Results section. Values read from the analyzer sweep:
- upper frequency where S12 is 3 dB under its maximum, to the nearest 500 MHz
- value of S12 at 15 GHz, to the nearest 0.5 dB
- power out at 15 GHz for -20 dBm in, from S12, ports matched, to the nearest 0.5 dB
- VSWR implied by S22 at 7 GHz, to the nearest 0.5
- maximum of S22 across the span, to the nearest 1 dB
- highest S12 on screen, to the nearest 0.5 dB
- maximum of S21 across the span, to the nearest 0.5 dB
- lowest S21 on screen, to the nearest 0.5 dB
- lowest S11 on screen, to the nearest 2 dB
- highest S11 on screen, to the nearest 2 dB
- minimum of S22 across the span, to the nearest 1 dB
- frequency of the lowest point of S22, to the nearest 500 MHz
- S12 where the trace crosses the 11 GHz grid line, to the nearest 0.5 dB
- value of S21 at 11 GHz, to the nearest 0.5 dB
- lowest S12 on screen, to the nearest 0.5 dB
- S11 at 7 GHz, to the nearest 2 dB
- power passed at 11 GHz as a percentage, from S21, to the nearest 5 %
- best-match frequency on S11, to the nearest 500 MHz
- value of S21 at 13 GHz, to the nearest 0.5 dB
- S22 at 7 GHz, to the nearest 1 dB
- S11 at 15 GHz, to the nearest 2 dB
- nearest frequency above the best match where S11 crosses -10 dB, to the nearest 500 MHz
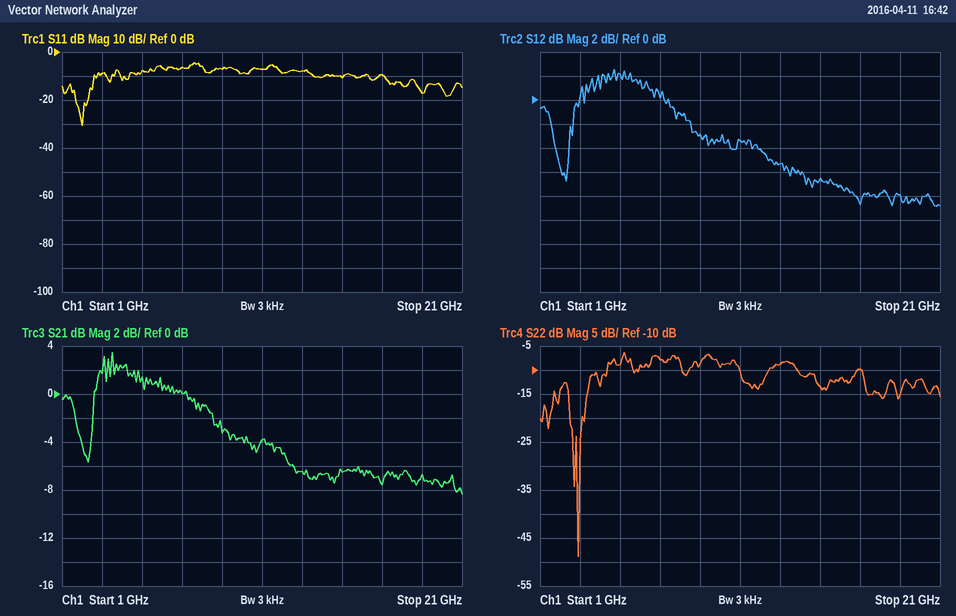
7.5 GHz
-6.5 dB
-26.5 dBm
2.5
-6 dB
2.5 dB
3.5 dB
-8.5 dB
-30 dB
-4 dB
-49 dB
3.0 GHz
-3.5 dB
-4.0 dB
-9.0 dB
-6 dB
40 %
2.0 GHz
-6.5 dB
-8 dB
-10 dB
2.5 GHz
